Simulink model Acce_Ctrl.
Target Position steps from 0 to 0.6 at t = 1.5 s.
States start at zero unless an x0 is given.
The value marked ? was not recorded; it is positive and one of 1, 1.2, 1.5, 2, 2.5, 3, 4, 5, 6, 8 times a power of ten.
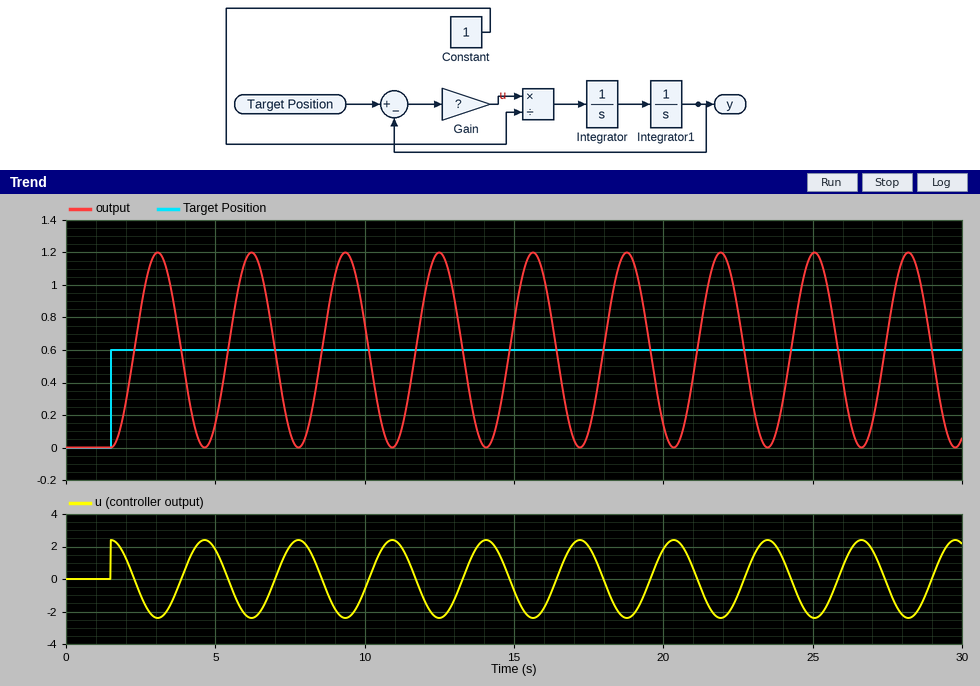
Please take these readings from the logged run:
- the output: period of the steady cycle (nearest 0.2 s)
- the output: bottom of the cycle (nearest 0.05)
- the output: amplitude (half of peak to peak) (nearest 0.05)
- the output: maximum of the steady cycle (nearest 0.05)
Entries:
3.2 s
0.00
0.60
1.20
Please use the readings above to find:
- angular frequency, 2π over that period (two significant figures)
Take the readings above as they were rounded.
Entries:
2.0 rad/s
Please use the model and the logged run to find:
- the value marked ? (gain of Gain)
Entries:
4
